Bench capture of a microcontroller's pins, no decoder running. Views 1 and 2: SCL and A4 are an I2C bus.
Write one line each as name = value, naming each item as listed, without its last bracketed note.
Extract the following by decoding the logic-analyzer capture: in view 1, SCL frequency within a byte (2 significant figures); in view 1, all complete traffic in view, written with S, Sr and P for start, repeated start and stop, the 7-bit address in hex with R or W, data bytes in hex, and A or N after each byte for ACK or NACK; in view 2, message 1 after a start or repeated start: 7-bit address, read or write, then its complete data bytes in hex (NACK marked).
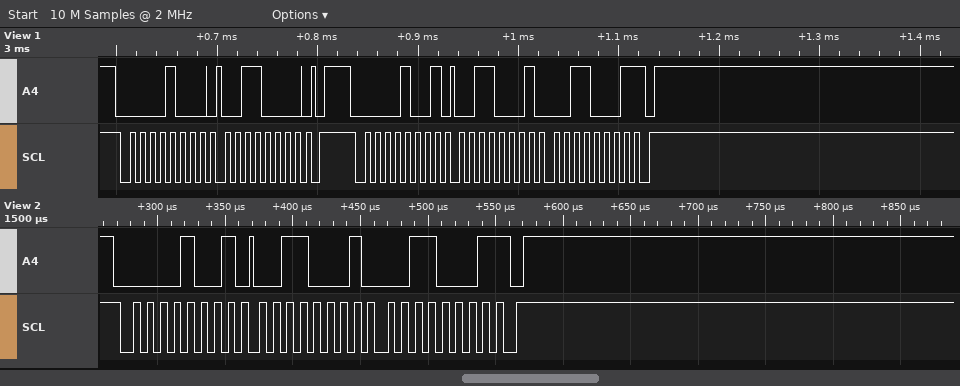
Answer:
in view 1, SCL frequency within a byte = 100 kHz
in view 1, all complete traffic in view, written with S, Sr and P for start, repeated start and stop, the 7-bit address in hex with R or W, data bytes in hex, and A or N after each byte for ACK or NACK = S 04W A 30 A P S 04R A 31 A 31 N P
in view 2, message 1 after a start or repeated start: 7-bit address, read or write, then its complete data bytes in hex = 0x04 read: 31 31 NACK
